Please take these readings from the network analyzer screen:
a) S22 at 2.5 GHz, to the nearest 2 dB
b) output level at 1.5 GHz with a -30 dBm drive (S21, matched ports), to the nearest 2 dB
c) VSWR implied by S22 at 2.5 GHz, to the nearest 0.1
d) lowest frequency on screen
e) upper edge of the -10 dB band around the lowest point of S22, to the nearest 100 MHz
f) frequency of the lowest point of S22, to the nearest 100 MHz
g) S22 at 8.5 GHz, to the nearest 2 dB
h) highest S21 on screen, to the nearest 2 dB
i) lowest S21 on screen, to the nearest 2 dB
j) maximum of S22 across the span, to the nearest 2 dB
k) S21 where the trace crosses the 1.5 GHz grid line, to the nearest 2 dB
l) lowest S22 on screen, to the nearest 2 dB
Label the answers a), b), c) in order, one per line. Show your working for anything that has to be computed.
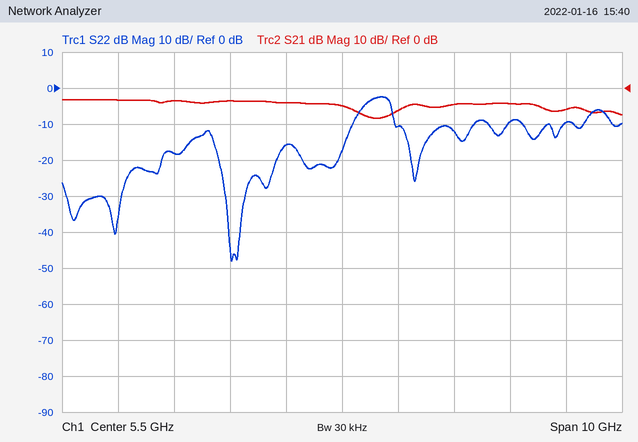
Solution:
a) -18 dB
b) -30 dBm + (-4 dB) = -34 dBm
c) |Γ| = 10^(-18/20) = 0.1259; VSWR = (1 + 0.1259)/(1 − 0.1259) ≈ 1.3
d) 500 MHz
e) 5.7 GHz
f) 3.5 GHz
g) -10 dB
h) -4 dB
i) -8 dB
j) -2 dB
k) -4 dB
l) -48 dB
